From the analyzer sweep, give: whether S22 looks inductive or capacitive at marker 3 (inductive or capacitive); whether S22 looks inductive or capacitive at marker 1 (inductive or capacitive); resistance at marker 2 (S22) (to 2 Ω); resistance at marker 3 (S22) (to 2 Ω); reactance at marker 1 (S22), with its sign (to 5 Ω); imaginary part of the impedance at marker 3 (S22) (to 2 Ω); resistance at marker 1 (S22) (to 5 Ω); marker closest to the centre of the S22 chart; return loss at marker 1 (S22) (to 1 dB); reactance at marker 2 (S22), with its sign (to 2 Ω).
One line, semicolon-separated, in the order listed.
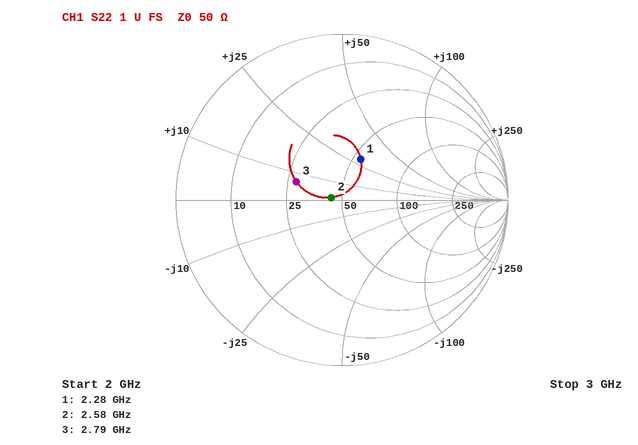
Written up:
inductive; inductive; 44 Ω; 28 Ω; +30 Ω; +6 Ω; 55 Ω; marker 2; 11 dB; +2 Ω
